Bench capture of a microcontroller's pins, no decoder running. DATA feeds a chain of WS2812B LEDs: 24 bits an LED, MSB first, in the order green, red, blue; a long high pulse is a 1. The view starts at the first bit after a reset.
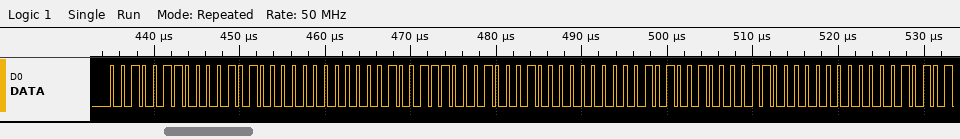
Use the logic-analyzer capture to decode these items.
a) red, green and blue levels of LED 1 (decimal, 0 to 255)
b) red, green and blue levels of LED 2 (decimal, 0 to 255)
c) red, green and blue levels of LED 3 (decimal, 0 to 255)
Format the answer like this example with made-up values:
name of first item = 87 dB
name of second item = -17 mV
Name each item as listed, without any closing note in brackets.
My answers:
red, green and blue levels of LED 1 = 20, 38, 0
red, green and blue levels of LED 2 = 17, 39, 0
red, green and blue levels of LED 3 = 12, 41, 0
